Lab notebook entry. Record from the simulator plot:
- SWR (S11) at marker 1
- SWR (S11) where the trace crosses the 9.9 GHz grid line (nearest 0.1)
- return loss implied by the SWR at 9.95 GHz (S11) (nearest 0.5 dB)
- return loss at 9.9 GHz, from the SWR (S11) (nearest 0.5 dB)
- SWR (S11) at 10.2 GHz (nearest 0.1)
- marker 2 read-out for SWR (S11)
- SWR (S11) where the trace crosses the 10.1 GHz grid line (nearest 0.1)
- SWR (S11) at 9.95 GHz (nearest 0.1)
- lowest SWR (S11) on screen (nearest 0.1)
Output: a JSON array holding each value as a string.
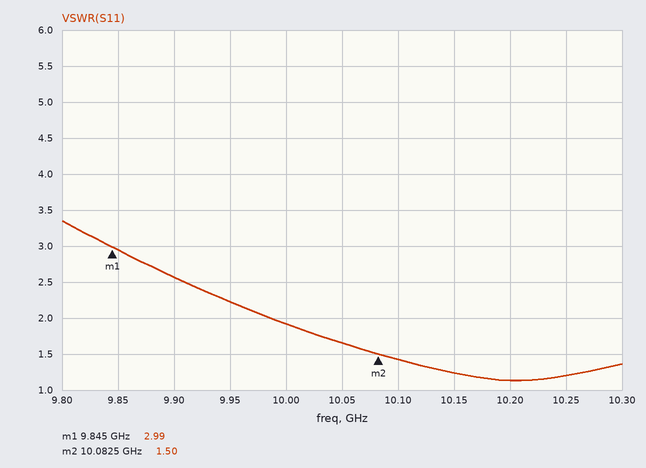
["2.99", "2.6", "8.5 dB", "7.0 dB", "1.1", "1.50", "1.4", "2.2", "1.1"]
